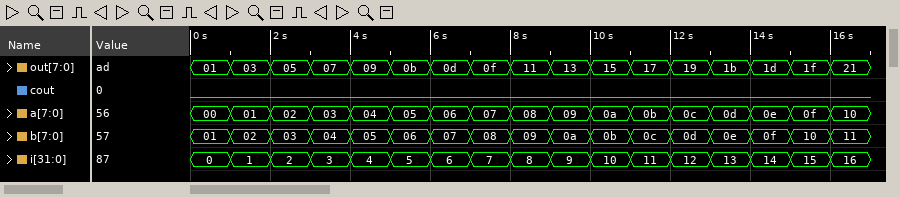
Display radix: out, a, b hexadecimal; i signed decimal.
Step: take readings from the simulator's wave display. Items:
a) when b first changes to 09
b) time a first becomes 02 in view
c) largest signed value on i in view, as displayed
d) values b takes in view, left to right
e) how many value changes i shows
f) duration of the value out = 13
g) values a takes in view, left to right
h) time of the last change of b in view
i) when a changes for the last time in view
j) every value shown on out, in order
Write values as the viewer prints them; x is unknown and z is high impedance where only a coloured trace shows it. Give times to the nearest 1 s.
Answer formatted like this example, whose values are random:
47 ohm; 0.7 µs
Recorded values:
8 s; 2 s; 16; 01, 02, 03, 04, 05, 06, 07, 08, 09, 0a, 0b, 0c, 0d, 0e, 0f, 10, 11; 16; 1 s; 00, 01, 02, 03, 04, 05, 06, 07, 08, 09, 0a, 0b, 0c, 0d, 0e, 0f, 10; 16 s; 16 s; 01, 03, 05, 07, 09, 0b, 0d, 0f, 11, 13, 15, 17, 19, 1b, 1d, 1f, 21
